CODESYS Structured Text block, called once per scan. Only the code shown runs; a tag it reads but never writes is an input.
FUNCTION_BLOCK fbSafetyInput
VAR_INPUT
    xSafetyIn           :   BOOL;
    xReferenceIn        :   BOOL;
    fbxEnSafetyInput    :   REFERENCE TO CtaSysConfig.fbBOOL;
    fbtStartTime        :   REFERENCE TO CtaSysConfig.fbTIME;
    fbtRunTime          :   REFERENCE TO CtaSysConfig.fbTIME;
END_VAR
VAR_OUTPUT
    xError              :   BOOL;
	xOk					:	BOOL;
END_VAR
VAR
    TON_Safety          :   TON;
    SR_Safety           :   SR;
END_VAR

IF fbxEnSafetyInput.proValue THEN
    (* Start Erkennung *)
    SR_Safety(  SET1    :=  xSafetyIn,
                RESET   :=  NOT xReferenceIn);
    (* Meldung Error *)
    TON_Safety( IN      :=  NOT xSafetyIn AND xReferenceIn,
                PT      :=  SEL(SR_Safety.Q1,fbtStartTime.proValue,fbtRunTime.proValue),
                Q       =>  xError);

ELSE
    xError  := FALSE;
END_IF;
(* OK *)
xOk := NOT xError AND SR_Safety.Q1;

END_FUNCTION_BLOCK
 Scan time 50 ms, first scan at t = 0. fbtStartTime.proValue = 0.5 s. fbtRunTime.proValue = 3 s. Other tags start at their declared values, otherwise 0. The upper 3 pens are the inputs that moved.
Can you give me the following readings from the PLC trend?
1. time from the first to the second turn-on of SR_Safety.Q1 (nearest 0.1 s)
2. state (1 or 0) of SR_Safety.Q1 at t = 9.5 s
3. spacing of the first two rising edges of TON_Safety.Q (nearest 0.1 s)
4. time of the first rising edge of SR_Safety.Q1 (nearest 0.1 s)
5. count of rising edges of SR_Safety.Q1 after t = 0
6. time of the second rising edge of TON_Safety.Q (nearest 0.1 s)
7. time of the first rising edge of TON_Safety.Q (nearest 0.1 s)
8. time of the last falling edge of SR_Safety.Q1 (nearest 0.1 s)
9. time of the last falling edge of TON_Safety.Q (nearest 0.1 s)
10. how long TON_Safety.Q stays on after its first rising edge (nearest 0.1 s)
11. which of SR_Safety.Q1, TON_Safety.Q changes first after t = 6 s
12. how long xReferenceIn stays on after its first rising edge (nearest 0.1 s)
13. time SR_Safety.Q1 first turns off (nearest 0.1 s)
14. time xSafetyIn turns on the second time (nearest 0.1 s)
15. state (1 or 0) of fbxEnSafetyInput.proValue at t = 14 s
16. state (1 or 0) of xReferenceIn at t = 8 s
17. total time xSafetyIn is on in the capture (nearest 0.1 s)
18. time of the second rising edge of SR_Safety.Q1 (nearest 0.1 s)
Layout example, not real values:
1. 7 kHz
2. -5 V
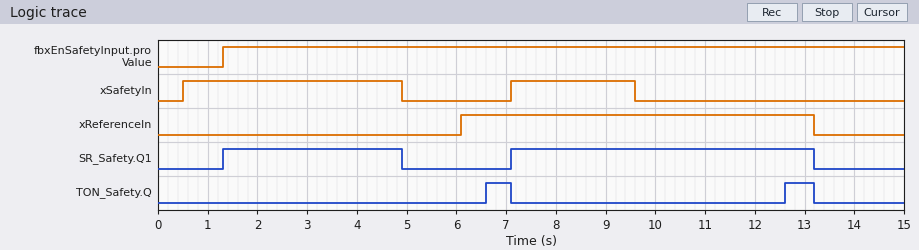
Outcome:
1. 5.8 s
2. 1
3. 6.0 s
4. 1.3 s
5. 2
6. 12.6 s
7. 6.6 s
8. 13.2 s
9. 13.2 s
10. 0.5 s
11. TON_Safety.Q
12. 7.1 s
13. 4.9 s
14. 7.1 s
15. 1
16. 1
17. 6.9 s
18. 7.1 s
